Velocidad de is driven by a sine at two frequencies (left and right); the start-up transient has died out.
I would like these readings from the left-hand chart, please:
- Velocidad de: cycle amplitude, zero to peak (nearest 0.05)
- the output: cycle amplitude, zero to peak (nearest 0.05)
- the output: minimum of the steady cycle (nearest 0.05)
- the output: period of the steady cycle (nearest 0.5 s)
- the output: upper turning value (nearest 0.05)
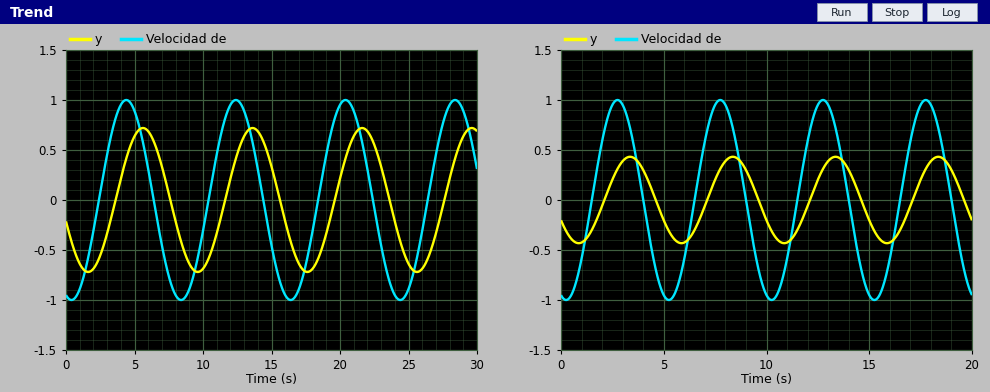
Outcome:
1.00
0.70
-0.70
8.0 s
0.70
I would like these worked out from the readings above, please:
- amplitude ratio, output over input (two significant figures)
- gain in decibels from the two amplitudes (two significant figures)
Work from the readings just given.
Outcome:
0.70
-3.1 dB
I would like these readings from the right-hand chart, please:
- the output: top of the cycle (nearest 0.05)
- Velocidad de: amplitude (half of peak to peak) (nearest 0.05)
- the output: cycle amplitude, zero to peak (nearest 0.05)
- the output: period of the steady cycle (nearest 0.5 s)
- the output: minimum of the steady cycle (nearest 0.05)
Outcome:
0.45
1.00
0.45
5.0 s
-0.45
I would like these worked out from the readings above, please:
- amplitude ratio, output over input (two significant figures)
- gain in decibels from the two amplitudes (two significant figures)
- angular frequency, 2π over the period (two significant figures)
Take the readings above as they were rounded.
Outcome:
0.45
-6.9 dB
1.3 rad/s
